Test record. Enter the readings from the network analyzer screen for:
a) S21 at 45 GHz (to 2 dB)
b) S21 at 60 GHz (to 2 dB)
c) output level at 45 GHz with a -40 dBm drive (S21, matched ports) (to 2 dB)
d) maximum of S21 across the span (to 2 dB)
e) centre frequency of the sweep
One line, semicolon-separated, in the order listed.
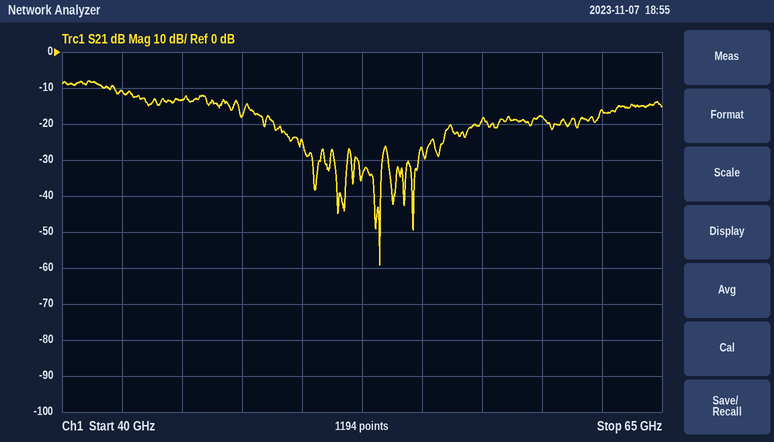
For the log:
-14 dB; -18 dB; -54 dBm; -8 dB; 52.5 GHz
